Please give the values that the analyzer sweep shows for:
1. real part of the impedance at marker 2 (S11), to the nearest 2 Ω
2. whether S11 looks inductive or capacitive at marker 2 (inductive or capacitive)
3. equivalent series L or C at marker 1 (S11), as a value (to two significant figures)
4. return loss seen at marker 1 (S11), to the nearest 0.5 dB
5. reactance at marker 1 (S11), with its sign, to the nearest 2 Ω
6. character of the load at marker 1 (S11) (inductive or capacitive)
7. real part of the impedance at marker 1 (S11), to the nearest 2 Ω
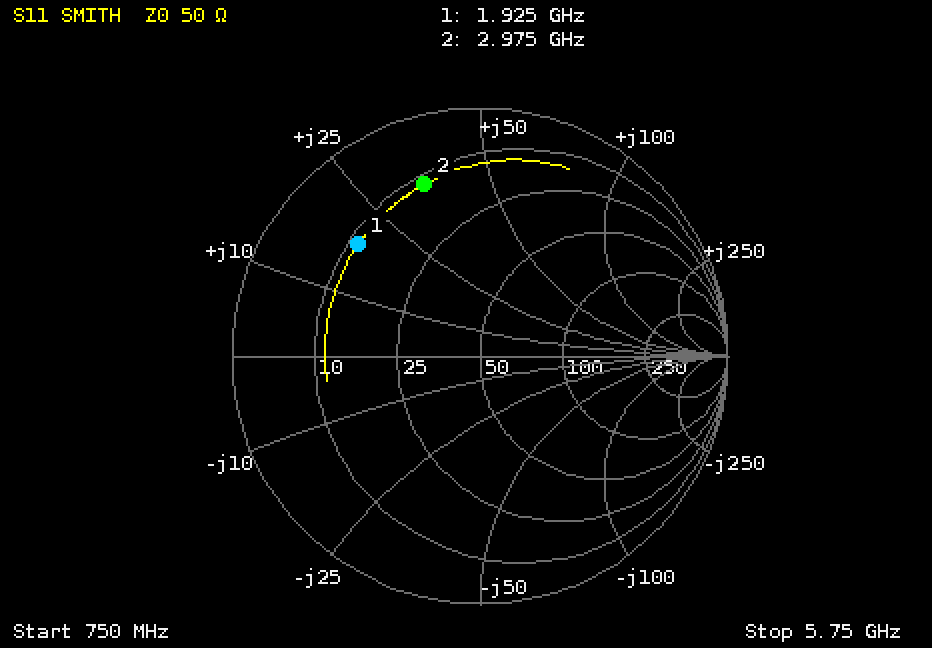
12 Ω
inductive
1.5 nH
3.5 dB
+18 Ω
inductive
12 Ω
